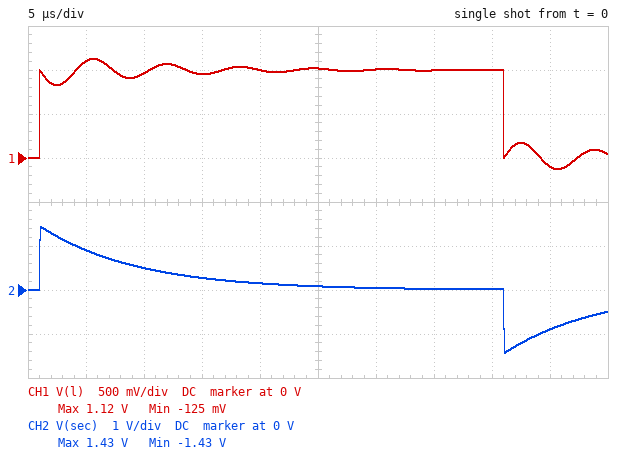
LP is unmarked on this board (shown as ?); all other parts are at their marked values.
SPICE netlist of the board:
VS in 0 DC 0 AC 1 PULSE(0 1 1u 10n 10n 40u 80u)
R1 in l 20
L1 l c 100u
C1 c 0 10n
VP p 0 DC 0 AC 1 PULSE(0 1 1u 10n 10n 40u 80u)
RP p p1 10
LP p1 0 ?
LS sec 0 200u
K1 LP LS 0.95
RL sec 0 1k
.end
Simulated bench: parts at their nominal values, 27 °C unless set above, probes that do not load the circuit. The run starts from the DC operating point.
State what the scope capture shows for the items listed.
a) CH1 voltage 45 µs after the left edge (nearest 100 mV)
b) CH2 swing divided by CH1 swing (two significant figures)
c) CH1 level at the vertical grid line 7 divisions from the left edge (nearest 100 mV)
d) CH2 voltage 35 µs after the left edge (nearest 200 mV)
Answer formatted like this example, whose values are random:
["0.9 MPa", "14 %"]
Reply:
["-100 mV", "2.3", "1.0 V", "0 V"]
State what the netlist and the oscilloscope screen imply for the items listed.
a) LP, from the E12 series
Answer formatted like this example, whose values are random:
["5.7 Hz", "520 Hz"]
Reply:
["82 µH"]
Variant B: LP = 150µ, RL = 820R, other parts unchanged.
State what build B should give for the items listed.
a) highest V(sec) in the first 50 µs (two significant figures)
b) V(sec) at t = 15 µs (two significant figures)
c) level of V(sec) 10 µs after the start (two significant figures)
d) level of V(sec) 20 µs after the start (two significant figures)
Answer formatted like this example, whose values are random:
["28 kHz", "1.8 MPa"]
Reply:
["1.1 V", "430 mV", "600 mV", "310 mV"]
